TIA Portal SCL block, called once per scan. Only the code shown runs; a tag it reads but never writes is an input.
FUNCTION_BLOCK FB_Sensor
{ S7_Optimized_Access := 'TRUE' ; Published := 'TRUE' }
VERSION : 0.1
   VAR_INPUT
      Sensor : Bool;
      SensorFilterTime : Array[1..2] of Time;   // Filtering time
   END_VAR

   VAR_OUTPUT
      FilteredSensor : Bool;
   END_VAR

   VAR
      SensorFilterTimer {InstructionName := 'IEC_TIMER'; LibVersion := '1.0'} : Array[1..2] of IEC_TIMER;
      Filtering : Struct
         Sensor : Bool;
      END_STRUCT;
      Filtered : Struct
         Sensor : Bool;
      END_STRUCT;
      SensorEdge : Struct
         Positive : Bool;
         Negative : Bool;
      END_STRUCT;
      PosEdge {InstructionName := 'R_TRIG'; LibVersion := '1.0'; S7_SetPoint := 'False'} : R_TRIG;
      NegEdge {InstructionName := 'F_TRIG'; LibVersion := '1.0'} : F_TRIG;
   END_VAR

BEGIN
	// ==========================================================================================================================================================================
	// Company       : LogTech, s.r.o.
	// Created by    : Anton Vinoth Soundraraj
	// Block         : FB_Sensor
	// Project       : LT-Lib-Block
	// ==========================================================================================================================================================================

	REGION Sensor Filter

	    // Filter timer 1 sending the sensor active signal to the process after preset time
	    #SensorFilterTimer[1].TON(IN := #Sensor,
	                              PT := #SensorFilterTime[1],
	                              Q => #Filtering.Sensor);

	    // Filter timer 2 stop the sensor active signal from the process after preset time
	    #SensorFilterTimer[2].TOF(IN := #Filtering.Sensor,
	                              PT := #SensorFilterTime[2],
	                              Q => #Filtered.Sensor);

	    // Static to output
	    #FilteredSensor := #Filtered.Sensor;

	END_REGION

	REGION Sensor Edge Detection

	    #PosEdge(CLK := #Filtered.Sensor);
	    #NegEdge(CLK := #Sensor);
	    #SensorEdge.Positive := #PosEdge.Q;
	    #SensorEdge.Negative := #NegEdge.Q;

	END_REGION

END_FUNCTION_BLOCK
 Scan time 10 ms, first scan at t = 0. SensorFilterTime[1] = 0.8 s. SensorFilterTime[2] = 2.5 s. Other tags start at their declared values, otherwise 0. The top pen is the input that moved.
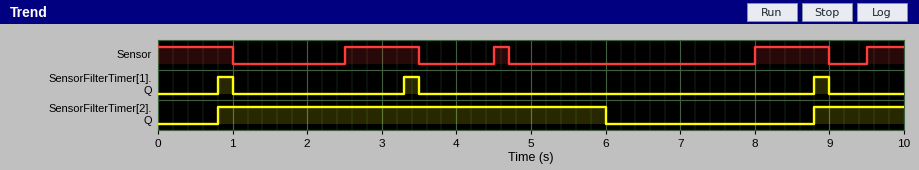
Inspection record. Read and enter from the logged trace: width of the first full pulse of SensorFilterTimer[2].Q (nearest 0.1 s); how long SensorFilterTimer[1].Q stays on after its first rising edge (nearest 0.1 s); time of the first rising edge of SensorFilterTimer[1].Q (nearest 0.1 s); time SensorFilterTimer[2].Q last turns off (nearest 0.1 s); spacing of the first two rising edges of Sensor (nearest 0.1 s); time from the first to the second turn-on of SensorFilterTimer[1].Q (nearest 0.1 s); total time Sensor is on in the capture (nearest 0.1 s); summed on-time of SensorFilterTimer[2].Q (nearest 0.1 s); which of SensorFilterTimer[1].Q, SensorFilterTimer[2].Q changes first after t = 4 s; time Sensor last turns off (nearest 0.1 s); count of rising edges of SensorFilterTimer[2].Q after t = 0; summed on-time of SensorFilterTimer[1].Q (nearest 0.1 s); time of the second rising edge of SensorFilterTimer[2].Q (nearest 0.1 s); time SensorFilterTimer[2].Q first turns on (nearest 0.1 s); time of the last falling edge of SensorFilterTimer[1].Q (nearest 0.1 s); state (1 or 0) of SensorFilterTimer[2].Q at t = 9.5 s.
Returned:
5.2 s
0.2 s
0.8 s
6.0 s
2.0 s
2.5 s
3.7 s
6.4 s
SensorFilterTimer[2].Q
9.0 s
2
0.6 s
8.8 s
0.8 s
9.0 s
1
